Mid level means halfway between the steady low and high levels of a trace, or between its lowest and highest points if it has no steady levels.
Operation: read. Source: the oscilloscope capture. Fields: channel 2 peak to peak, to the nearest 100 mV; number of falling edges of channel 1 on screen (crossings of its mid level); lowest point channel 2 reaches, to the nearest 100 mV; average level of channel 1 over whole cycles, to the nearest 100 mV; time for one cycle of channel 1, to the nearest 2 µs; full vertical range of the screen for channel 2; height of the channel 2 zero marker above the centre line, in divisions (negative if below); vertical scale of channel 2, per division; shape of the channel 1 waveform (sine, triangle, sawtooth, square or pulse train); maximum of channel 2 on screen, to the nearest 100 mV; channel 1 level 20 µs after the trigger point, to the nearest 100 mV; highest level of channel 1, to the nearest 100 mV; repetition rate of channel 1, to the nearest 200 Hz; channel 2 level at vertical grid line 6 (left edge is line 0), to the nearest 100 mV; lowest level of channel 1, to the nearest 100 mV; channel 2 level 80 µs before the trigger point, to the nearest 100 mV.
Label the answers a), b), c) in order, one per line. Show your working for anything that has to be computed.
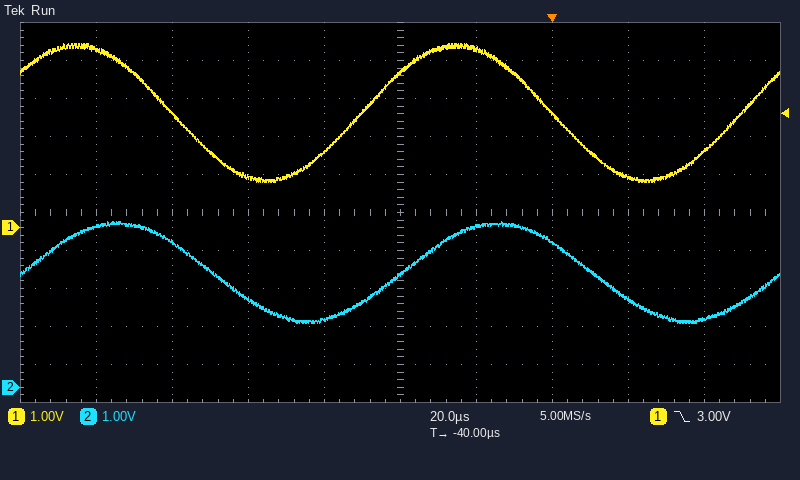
a) 4.4 V − (1.7 V) = 2.7 V
b) 2
c) 1.7 V
d) (4.8 V + (1.2 V)) / 2 ≈ 3.0 V
e) 100 µs
f) 10 V
g) -4.6 div
h) 1 V
i) sine
j) 4.4 V
k) 1.3 V
l) 4.8 V
m) 1 / 100 µs ≈ 10.0 kHz
n) 4.2 V
o) 1.2 V
p) 2.3 V
